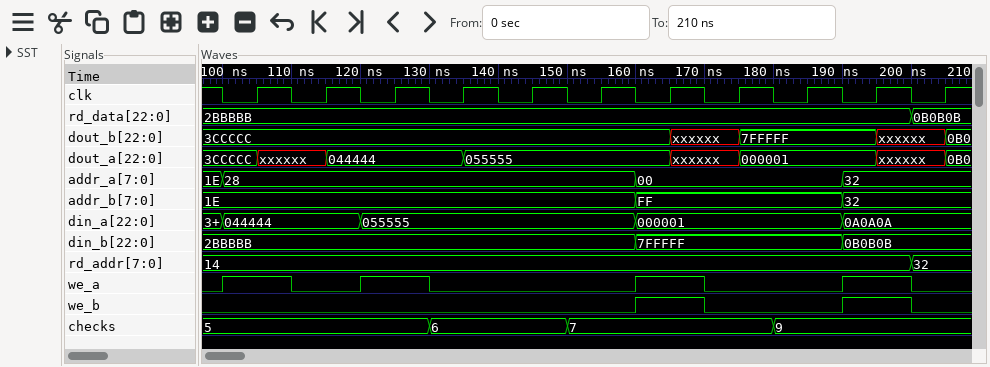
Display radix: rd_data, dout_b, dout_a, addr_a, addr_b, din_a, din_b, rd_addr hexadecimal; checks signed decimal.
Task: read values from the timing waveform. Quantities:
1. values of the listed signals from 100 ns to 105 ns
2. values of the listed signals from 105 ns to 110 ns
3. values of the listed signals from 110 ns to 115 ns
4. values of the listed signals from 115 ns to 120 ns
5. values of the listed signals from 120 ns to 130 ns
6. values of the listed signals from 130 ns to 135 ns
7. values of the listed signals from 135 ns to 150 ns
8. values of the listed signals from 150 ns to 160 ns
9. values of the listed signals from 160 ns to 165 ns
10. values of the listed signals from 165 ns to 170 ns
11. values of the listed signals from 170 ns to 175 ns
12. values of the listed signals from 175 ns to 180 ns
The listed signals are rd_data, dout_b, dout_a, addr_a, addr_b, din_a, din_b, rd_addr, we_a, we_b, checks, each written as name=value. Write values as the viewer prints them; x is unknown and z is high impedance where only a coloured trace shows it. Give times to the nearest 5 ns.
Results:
rd_data=2BBBBB, dout_b=3CCCCC, dout_a=3CCCCC, addr_a=28, addr_b=1E, din_a=044444, din_b=2BBBBB, rd_addr=14, we_a=1, we_b=0, checks=5
rd_data=2BBBBB, dout_b=3CCCCC, dout_a=xxxxxx, addr_a=28, addr_b=1E, din_a=044444, din_b=2BBBBB, rd_addr=14, we_a=1, we_b=0, checks=5
rd_data=2BBBBB, dout_b=3CCCCC, dout_a=xxxxxx, addr_a=28, addr_b=1E, din_a=044444, din_b=2BBBBB, rd_addr=14, we_a=0, we_b=0, checks=5
rd_data=2BBBBB, dout_b=3CCCCC, dout_a=044444, addr_a=28, addr_b=1E, din_a=044444, din_b=2BBBBB, rd_addr=14, we_a=0, we_b=0, checks=5
rd_data=2BBBBB, dout_b=3CCCCC, dout_a=044444, addr_a=28, addr_b=1E, din_a=055555, din_b=2BBBBB, rd_addr=14, we_a=1, we_b=0, checks=5
rd_data=2BBBBB, dout_b=3CCCCC, dout_a=044444, addr_a=28, addr_b=1E, din_a=055555, din_b=2BBBBB, rd_addr=14, we_a=0, we_b=0, checks=6
rd_data=2BBBBB, dout_b=3CCCCC, dout_a=055555, addr_a=28, addr_b=1E, din_a=055555, din_b=2BBBBB, rd_addr=14, we_a=0, we_b=0, checks=6
rd_data=2BBBBB, dout_b=3CCCCC, dout_a=055555, addr_a=28, addr_b=1E, din_a=055555, din_b=2BBBBB, rd_addr=14, we_a=0, we_b=0, checks=7
rd_data=2BBBBB, dout_b=3CCCCC, dout_a=055555, addr_a=00, addr_b=FF, din_a=000001, din_b=7FFFFF, rd_addr=14, we_a=1, we_b=1, checks=7
rd_data=2BBBBB, dout_b=xxxxxx, dout_a=xxxxxx, addr_a=00, addr_b=FF, din_a=000001, din_b=7FFFFF, rd_addr=14, we_a=1, we_b=1, checks=7
rd_data=2BBBBB, dout_b=xxxxxx, dout_a=xxxxxx, addr_a=00, addr_b=FF, din_a=000001, din_b=7FFFFF, rd_addr=14, we_a=0, we_b=0, checks=7
rd_data=2BBBBB, dout_b=7FFFFF, dout_a=000001, addr_a=00, addr_b=FF, din_a=000001, din_b=7FFFFF, rd_addr=14, we_a=0, we_b=0, checks=7
